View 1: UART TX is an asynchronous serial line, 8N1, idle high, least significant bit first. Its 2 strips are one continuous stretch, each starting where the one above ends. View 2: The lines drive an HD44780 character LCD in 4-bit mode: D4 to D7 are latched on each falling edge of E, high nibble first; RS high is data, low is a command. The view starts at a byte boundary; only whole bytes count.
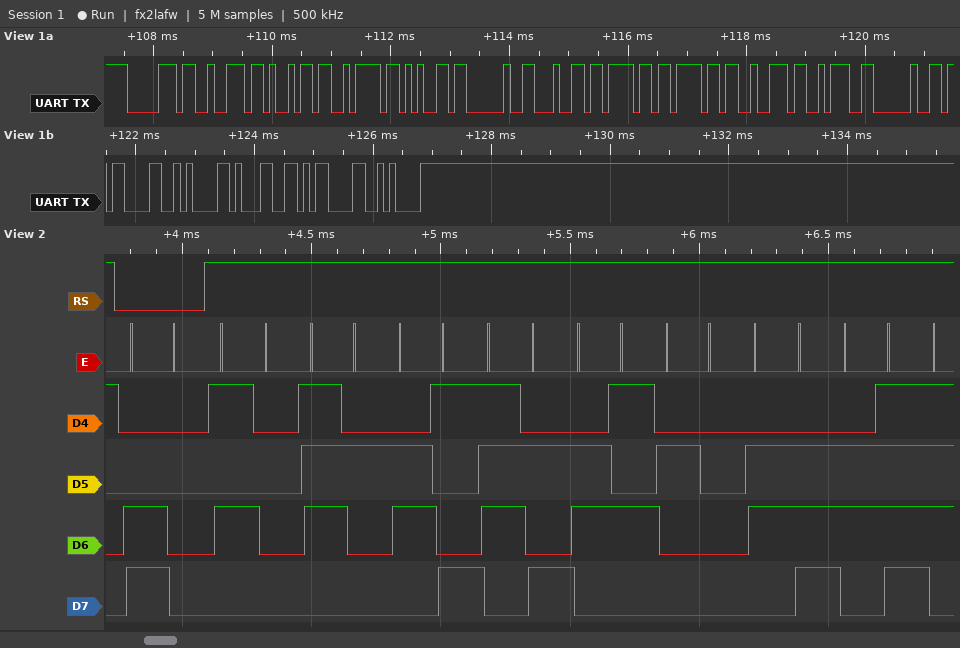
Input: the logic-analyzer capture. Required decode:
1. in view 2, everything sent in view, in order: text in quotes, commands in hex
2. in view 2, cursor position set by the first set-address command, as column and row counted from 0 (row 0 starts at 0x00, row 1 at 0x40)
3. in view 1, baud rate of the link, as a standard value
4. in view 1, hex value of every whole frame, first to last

0xC0 "Prize no"
column 0, row 1
9600 baud
0x70 0x72 0x69 0x7A 0x65 0x20 0x64 0x6F 0x6F 0x72 0x3A 0x20 0x0D 0x0A 0x31 0x0D 0x0A
